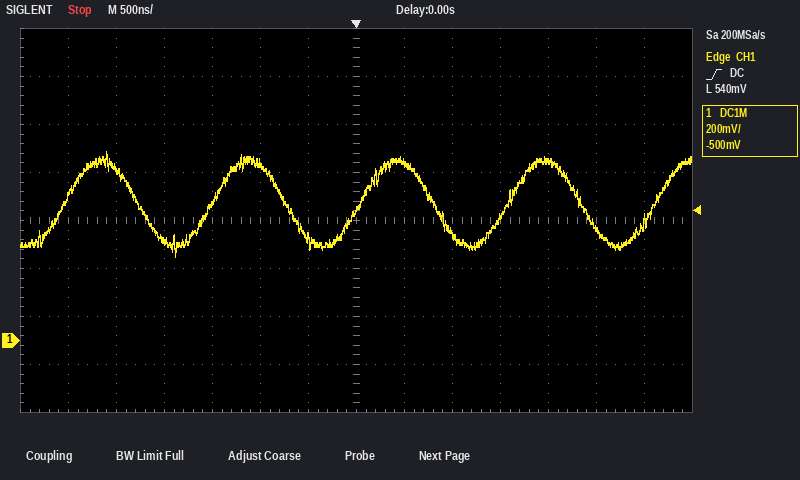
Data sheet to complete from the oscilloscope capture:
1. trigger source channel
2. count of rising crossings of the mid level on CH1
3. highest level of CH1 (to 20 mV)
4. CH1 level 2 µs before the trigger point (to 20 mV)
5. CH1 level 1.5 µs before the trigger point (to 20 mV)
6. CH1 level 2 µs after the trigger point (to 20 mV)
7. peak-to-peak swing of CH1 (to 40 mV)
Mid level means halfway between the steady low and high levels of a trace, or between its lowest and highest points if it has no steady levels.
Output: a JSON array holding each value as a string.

["CH1", "5", "780 mV", "420 mV", "580 mV", "740 mV", "440 mV"]
